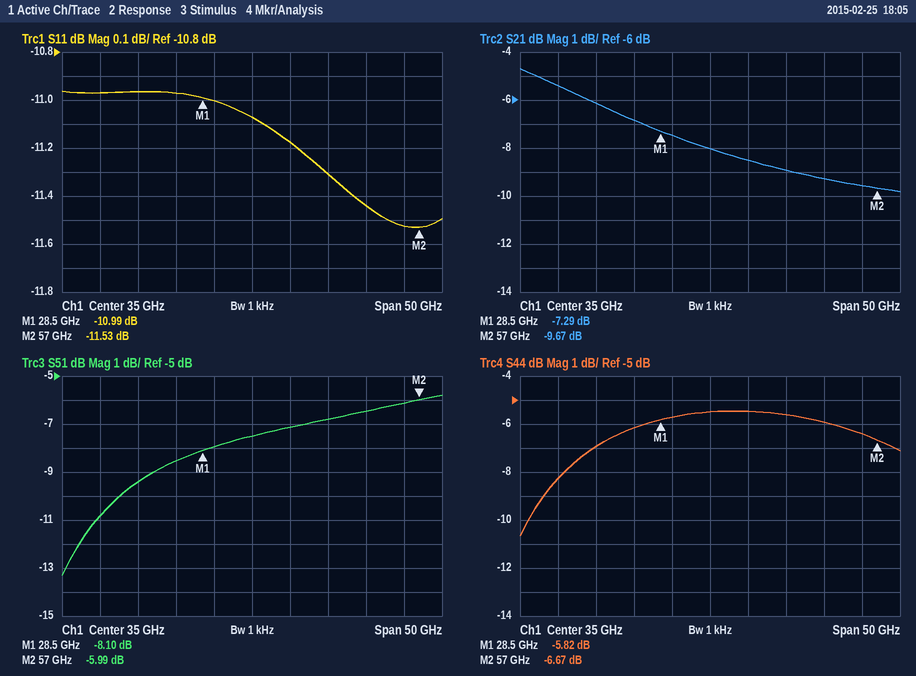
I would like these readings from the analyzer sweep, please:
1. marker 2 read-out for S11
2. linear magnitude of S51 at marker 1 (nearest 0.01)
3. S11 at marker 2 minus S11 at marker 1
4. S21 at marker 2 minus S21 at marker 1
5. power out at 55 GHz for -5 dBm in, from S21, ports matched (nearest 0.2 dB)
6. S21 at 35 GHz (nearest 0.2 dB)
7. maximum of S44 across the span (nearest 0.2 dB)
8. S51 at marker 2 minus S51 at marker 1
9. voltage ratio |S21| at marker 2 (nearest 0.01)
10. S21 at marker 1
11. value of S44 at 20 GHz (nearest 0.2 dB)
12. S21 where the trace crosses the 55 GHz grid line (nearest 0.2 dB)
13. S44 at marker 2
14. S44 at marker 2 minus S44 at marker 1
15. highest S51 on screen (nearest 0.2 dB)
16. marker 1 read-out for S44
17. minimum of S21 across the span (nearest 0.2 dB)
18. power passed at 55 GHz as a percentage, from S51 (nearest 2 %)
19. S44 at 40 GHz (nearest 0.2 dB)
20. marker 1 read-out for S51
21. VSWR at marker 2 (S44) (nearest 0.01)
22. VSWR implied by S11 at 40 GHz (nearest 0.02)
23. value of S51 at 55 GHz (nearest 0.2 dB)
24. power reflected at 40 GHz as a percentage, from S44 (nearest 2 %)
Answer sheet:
-11.53 dB
0.39
-0.54 dB
-2.38 dB
-14.6 dBm
-8.0 dB
-5.4 dB
2.11 dB
0.33
-7.29 dB
-7.0 dB
-9.6 dB
-6.67 dB
-0.85 dB
-5.8 dB
-5.82 dB
-9.8 dB
24 %
-5.4 dB
-8.10 dB
2.73
1.76
-6.2 dB
28 %
